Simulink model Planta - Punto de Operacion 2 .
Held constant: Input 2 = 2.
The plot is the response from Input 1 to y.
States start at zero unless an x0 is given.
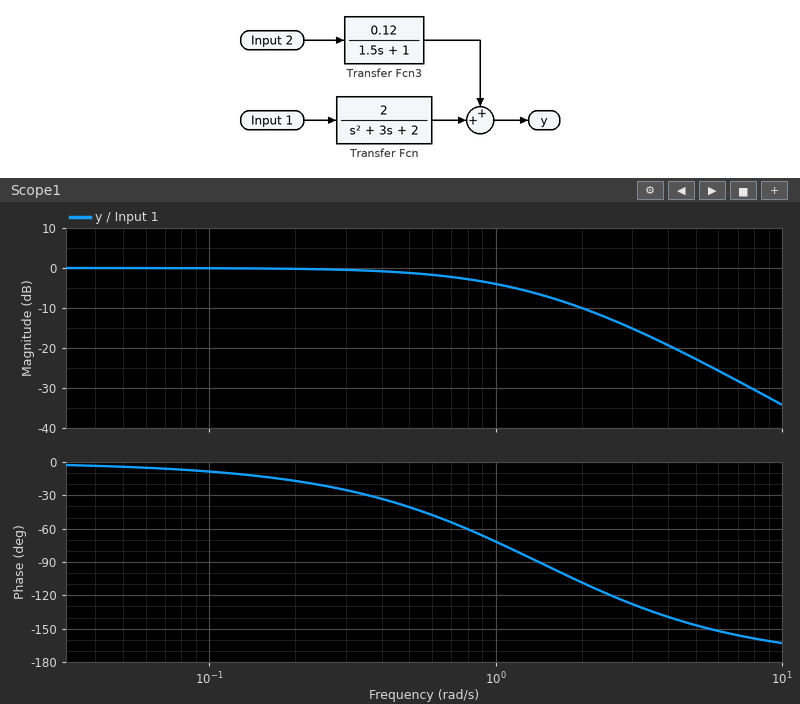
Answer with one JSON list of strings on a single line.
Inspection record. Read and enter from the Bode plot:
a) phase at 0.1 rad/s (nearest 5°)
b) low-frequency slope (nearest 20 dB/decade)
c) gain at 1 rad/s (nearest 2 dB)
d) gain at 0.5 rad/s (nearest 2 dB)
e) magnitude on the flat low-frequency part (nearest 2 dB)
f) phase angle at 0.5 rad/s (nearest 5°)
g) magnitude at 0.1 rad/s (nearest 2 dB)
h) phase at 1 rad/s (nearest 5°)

["-10°", "0 dB/decade", "-4 dB", "-2 dB", "0 dB", "-40°", "0 dB", "-70°"]
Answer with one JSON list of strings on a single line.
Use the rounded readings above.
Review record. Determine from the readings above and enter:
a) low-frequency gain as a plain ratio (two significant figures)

["1.0"]
